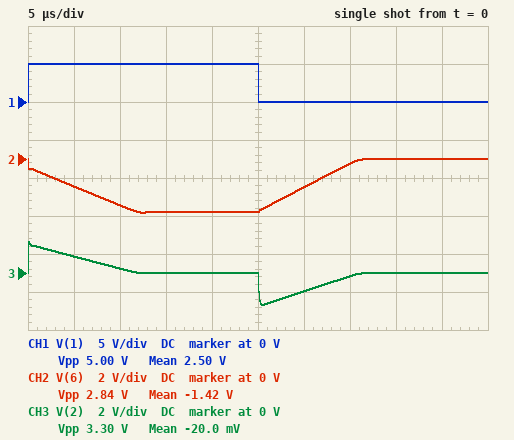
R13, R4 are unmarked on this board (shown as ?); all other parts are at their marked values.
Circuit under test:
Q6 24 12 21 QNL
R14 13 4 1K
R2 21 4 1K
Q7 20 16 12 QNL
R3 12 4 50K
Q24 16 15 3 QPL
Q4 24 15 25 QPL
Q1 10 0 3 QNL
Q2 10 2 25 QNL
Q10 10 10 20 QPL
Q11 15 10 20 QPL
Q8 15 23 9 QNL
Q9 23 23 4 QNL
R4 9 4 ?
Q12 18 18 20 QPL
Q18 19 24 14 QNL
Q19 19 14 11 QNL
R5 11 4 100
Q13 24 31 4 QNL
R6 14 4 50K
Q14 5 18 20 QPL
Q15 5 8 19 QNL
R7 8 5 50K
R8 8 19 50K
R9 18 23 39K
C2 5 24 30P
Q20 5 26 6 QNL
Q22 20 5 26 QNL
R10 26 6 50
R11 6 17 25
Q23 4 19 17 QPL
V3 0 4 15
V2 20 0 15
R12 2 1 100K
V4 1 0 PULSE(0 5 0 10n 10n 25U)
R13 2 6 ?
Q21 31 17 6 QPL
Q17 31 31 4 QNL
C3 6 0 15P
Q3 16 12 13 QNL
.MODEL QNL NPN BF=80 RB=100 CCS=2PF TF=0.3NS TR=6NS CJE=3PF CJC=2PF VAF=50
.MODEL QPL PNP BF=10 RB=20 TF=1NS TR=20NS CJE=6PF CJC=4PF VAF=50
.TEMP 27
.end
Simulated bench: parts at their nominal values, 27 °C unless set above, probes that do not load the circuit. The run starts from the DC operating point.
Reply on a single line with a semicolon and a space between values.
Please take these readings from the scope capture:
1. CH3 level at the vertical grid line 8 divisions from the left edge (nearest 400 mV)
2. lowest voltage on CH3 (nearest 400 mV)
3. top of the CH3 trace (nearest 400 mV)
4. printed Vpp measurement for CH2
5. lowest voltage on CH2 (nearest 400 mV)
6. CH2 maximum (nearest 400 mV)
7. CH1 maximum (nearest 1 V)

0 V; -1.6 V; 1.6 V; 2.84 V; -2.8 V; 0 V; 5 V
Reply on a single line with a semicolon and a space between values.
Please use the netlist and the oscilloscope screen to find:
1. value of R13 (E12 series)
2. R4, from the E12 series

56 kΩ; 12 kΩ
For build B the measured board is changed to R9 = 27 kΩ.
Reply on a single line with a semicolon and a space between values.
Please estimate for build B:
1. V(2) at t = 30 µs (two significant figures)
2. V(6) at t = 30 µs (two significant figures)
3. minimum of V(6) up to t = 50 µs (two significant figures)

-910 mV; -1.4 V; -2.8 V
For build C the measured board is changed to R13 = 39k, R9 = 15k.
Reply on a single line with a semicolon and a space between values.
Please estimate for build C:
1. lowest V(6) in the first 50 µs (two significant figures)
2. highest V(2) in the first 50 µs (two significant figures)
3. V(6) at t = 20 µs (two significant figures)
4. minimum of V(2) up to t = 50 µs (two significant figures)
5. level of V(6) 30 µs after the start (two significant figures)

-2.0 V; 1.3 V; -1.9 V; -1.3 V; -390 mV
